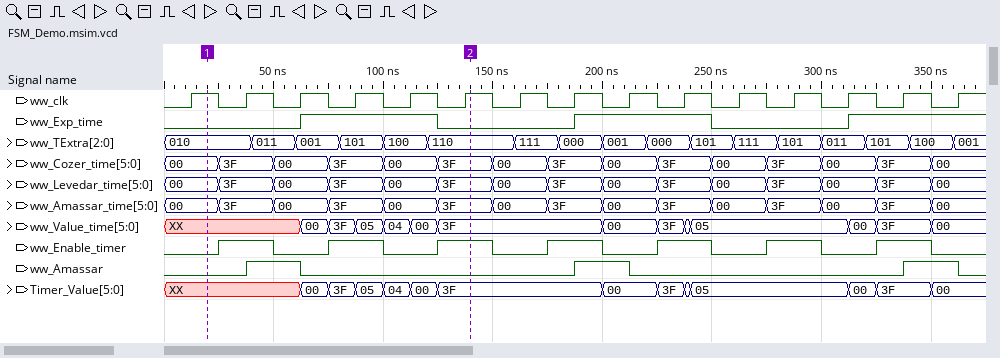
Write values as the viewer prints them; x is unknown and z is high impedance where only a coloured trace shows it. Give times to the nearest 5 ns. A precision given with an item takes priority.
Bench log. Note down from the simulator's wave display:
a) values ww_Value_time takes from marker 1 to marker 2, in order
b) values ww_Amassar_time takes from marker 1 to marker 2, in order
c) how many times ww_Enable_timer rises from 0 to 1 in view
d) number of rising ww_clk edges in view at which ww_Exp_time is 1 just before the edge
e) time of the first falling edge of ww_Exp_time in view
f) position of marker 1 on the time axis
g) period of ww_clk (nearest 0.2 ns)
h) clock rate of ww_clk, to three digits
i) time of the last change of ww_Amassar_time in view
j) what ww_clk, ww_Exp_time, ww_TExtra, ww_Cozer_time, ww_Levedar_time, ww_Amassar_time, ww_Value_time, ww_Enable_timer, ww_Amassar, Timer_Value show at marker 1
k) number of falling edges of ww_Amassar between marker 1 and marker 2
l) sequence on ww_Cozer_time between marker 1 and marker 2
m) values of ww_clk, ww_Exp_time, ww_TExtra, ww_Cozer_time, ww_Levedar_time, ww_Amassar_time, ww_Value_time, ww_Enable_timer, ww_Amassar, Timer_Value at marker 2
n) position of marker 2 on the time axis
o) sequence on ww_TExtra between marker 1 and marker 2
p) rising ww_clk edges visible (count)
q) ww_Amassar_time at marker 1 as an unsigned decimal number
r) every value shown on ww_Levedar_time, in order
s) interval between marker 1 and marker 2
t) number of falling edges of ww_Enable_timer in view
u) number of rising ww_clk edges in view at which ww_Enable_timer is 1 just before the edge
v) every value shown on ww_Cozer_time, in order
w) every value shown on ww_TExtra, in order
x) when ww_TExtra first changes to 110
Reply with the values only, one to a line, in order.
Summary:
XX, 00, 3F, 05, 04, 00, 3F
00, 3F, 00, 3F, 00, 3F
7
6
125 ns
20 ns
25 ns
40.0 MHz
350 ns
ww_clk=1, ww_Exp_time=0, ww_TExtra=010, ww_Cozer_time=00, ww_Levedar_time=00, ww_Amassar_time=00, ww_Value_time=XX, ww_Enable_timer=0, ww_Amassar=0, Timer_Value=XX
1
00, 3F, 00, 3F, 00, 3F
ww_clk=1, ww_Exp_time=0, ww_TExtra=110, ww_Cozer_time=3F, ww_Levedar_time=3F, ww_Amassar_time=3F, ww_Value_time=3F, ww_Enable_timer=1, ww_Amassar=0, Timer_Value=3F
140 ns
010, 011, 001, 101, 100, 110
15
0
00, 3F, 00, 3F, 00, 3F, 00, 3F, 00, 3F, 00, 3F, 00, 3F, 00
120 ns
7
7
00, 3F, 00, 3F, 00, 3F, 00, 3F, 00, 3F, 00, 3F, 00, 3F, 00
010, 011, 001, 101, 100, 110, 111, 000, 001, 000, 101, 111, 101, 011, 101, 100, 001
120 ns
